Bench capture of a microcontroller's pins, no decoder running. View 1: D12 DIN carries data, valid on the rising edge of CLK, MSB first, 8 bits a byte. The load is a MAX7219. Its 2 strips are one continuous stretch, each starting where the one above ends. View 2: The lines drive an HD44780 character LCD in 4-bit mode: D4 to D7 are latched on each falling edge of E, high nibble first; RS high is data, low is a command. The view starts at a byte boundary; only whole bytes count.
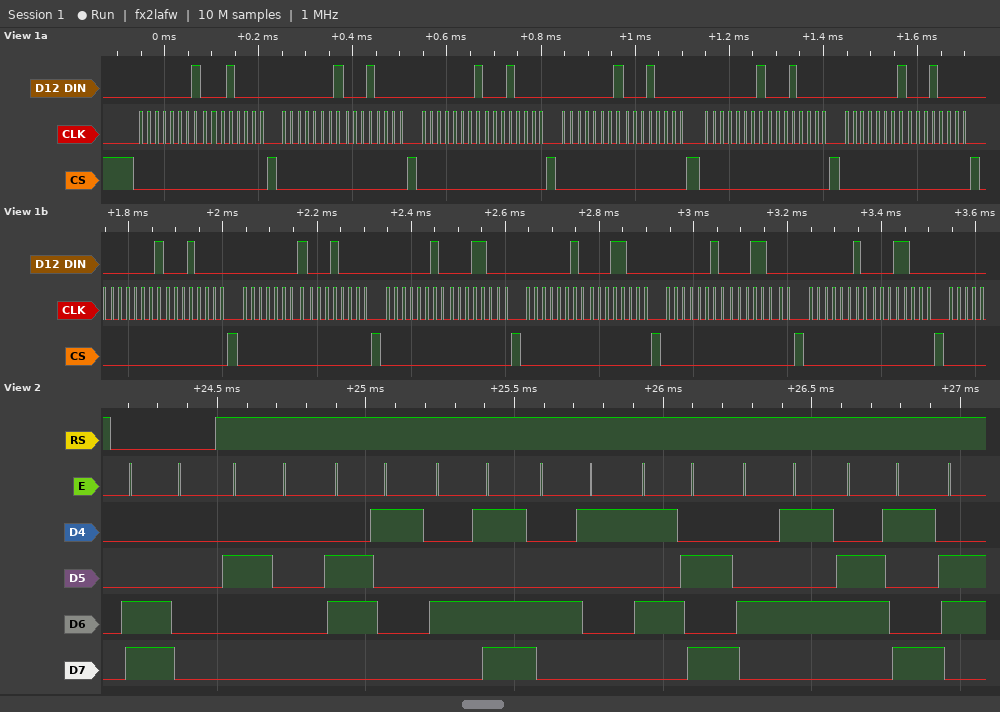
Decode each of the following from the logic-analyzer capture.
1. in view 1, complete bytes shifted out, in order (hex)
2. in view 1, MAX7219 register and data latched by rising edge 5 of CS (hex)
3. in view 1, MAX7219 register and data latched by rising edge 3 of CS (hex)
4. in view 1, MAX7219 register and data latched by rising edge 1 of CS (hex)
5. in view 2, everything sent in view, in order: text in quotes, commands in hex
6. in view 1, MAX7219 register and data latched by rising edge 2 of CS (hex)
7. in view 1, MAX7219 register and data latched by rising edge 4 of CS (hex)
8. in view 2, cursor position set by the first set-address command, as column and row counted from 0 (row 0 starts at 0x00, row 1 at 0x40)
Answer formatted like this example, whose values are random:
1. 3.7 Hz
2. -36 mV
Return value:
1. 01 10 01 10 01 10 01 10 01 10 01 10 01 10 01 10 02 18 02 18 02 18 02 18
2. register 0x1, data 0x10
3. register 0x1, data 0x10
4. register 0x1, data 0x10
5. 0xC0 " aMAZEi"
6. register 0x1, data 0x10
7. register 0x1, data 0x10
8. column 0, row 1
